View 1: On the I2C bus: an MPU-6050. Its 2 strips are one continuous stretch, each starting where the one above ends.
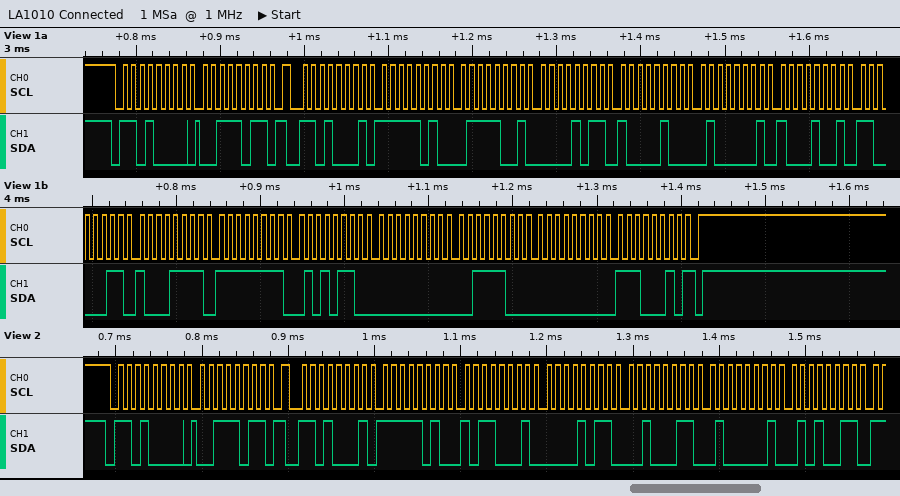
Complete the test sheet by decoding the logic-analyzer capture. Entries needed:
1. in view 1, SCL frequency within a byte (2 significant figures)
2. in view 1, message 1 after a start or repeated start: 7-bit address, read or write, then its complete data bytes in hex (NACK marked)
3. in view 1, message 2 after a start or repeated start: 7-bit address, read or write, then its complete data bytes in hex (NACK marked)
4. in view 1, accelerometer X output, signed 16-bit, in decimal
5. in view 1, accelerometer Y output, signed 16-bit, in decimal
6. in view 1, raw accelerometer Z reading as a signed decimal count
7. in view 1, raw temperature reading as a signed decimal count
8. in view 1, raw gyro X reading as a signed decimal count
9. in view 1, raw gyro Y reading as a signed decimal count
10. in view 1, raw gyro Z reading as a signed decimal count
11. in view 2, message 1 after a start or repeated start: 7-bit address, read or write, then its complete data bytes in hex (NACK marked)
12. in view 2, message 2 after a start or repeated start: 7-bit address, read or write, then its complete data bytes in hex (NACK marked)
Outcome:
100 kHz
0x68 write: 3B
0x68 read: FA 79 0B 84 41 89 C3 8F FF 56 00 3C 00 E2 NACK
-1415
2948
16777
-15473
-170
60
226
0x68 write: 3B
0x68 read: FA B1 0B 23 41 53
